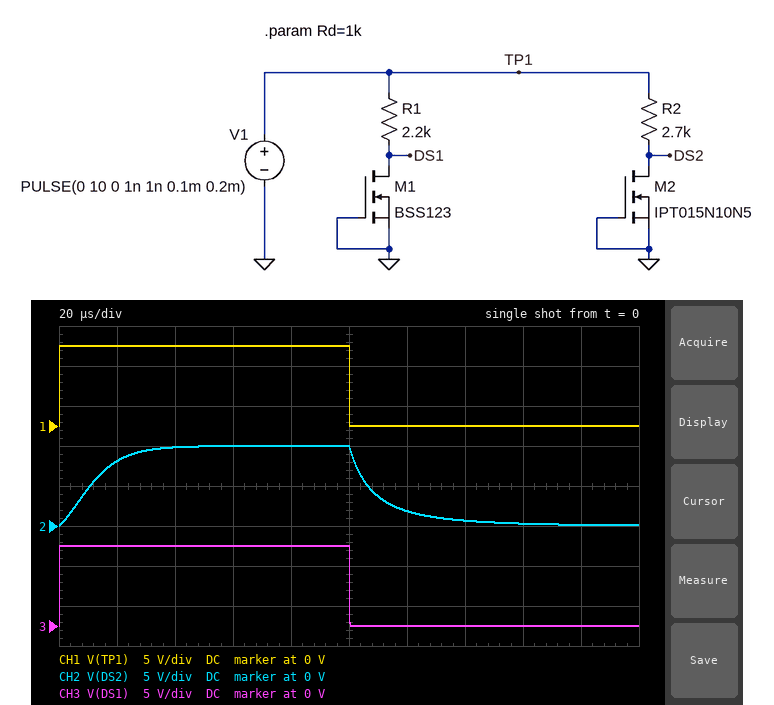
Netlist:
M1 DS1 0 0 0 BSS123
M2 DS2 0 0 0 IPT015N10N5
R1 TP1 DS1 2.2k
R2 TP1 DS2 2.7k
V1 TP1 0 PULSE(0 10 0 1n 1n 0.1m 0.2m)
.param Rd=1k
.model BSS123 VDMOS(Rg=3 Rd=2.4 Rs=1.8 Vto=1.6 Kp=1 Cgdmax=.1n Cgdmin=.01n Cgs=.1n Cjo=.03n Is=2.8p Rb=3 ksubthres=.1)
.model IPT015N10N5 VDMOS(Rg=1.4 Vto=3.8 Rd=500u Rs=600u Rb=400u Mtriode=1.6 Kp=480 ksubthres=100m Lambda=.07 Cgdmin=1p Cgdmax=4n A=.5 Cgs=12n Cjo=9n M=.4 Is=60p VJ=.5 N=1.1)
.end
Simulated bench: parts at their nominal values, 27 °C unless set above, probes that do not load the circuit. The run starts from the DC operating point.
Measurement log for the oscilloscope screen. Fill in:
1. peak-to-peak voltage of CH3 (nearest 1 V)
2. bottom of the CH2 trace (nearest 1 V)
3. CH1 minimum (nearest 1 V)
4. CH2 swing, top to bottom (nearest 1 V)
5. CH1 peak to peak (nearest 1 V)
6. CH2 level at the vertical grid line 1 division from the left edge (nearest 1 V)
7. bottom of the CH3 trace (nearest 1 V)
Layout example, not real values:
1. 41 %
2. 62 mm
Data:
1. 10 V
2. 0 V
3. 0 V
4. 10 V
5. 10 V
6. 8 V
7. 0 V
